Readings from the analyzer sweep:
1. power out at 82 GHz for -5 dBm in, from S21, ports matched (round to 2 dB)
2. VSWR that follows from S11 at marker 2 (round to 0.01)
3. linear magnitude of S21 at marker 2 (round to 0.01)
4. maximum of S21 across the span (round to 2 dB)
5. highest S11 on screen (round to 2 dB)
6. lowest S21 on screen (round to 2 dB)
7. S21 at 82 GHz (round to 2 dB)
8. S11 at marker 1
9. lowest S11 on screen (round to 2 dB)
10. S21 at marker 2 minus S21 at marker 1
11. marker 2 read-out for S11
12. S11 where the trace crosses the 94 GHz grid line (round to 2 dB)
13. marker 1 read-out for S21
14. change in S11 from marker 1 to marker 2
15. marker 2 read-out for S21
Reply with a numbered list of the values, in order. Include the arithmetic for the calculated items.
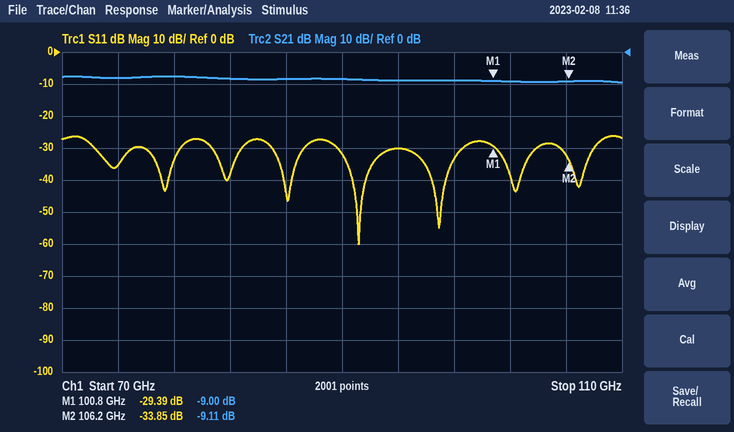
1. -5 dBm + (-8 dB) = -14 dBm
2. (1 + 0.0203)/(1 − 0.0203) ≈ 1.04
3. 10^(-9.11/20) ≈ 0.35
4. -8 dB
5. -26 dB
6. -10 dB
7. -8 dB
8. -29.39 dB
9. -60 dB
10. -9.11 − (-9) = -0.11 dB
11. -33.85 dB
12. -30 dB
13. -9.00 dB
14. -33.85 − (-29.39) = -4.46 dB
15. -9.11 dB
